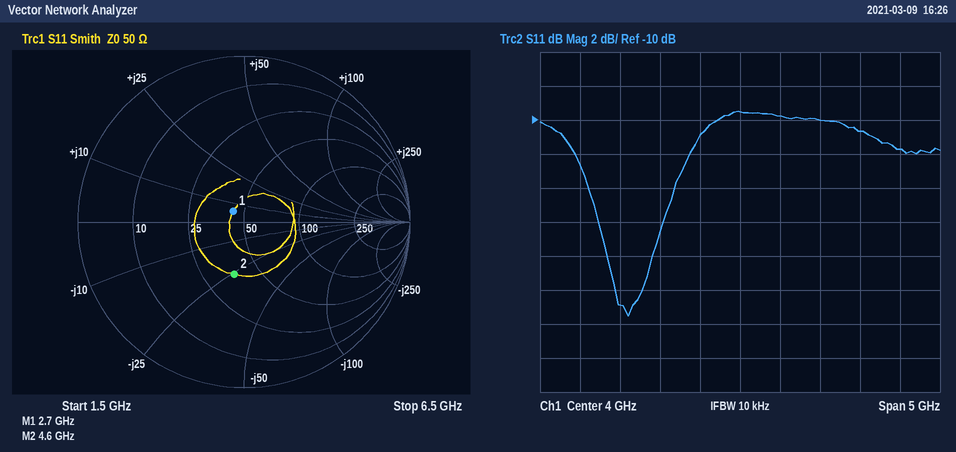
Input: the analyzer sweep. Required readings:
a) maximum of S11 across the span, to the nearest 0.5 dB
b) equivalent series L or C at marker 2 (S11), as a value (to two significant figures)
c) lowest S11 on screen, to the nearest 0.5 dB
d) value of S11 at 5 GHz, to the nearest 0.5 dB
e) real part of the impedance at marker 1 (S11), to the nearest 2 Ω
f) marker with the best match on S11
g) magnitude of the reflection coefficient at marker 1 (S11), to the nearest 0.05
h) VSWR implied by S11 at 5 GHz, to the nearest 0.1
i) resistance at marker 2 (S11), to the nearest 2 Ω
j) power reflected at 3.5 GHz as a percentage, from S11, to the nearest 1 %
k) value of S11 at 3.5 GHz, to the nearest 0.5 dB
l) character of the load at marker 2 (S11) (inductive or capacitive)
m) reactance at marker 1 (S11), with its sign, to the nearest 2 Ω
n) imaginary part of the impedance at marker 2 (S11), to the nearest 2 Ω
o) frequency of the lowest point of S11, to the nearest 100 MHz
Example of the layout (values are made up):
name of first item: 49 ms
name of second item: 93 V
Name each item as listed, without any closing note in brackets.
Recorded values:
maximum of S11 across the span, to the nearest 0.5 dB: -9.5 dB
equivalent series L or C at marker 2 (S11), as a value: 1.3 pF
lowest S11 on screen, to the nearest 0.5 dB: -21.5 dB
value of S11 at 5 GHz, to the nearest 0.5 dB: -10.0 dB
real part of the impedance at marker 1 (S11), to the nearest 2 Ω: 44 Ω
marker with the best match on S11: marker 1
magnitude of the reflection coefficient at marker 1 (S11), to the nearest 0.05: 0.10
VSWR implied by S11 at 5 GHz, to the nearest 0.1: 1.9
resistance at marker 2 (S11), to the nearest 2 Ω: 36 Ω
power reflected at 3.5 GHz as a percentage, from S11, to the nearest 1 %: 8 %
value of S11 at 3.5 GHz, to the nearest 0.5 dB: -11.0 dB
character of the load at marker 2 (S11): capacitive
reactance at marker 1 (S11), with its sign, to the nearest 2 Ω: +6 Ω
imaginary part of the impedance at marker 2 (S11), to the nearest 2 Ω: -26 Ω
frequency of the lowest point of S11, to the nearest 100 MHz: 2.6 GHz
